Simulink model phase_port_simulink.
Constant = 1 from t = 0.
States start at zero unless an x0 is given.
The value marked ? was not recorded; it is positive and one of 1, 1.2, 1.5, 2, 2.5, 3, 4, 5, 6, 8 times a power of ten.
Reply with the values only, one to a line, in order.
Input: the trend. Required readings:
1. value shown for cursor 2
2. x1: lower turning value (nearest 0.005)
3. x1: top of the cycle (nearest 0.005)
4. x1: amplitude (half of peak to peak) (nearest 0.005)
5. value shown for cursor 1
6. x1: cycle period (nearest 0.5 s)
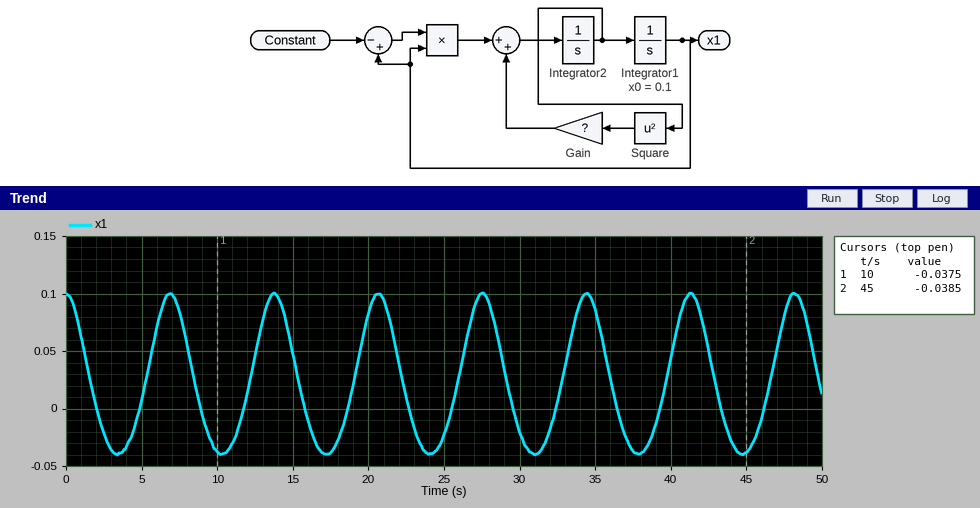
-0.0385
-0.040
0.100
0.070
-0.0375
7.0 s
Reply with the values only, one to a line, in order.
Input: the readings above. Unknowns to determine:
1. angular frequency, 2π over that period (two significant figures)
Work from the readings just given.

0.90 rad/s
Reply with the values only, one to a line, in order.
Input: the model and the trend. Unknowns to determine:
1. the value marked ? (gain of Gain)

10
